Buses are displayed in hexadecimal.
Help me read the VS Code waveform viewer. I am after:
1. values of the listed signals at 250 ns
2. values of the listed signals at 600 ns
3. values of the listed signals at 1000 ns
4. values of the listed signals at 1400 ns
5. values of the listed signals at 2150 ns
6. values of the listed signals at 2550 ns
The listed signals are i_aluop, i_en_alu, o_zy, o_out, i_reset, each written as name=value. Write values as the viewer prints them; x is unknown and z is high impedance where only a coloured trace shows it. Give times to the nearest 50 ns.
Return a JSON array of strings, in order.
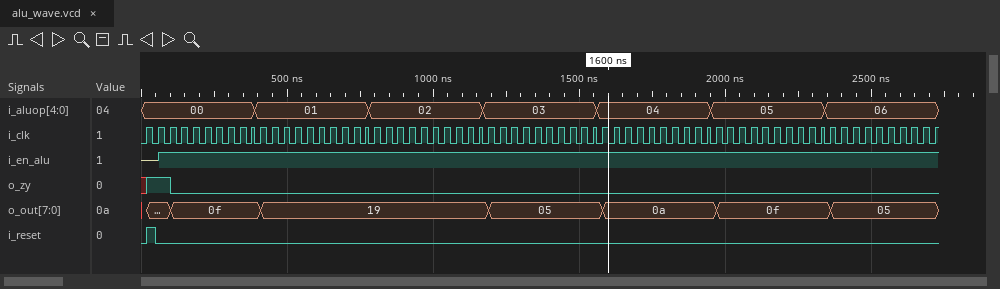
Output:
["i_aluop=00, i_en_alu=1, o_zy=0, o_out=0f, i_reset=0", "i_aluop=01, i_en_alu=1, o_zy=0, o_out=19, i_reset=0", "i_aluop=02, i_en_alu=1, o_zy=0, o_out=19, i_reset=0", "i_aluop=03, i_en_alu=1, o_zy=0, o_out=05, i_reset=0", "i_aluop=05, i_en_alu=1, o_zy=0, o_out=0f, i_reset=0", "i_aluop=06, i_en_alu=1, o_zy=0, o_out=05, i_reset=0"]
